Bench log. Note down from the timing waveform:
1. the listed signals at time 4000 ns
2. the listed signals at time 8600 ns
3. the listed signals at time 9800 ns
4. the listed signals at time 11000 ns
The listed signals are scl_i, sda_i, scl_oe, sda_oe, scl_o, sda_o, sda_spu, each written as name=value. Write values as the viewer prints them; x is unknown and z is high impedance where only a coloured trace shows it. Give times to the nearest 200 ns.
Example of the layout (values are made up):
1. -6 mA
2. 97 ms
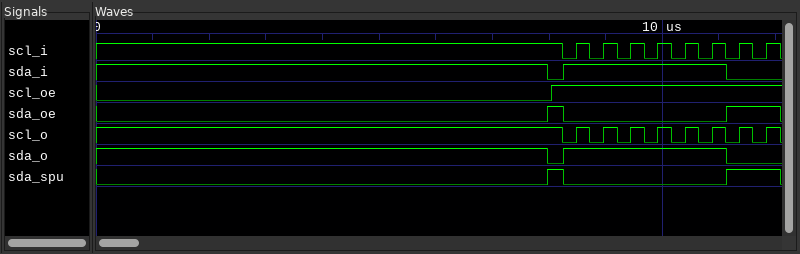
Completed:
1. scl_i=1, sda_i=1, scl_oe=0, sda_oe=0, scl_o=1, sda_o=1, sda_spu=0
2. scl_i=1, sda_i=1, scl_oe=1, sda_oe=0, scl_o=1, sda_o=1, sda_spu=0
3. scl_i=0, sda_i=1, scl_oe=1, sda_oe=0, scl_o=0, sda_o=1, sda_spu=0
4. scl_i=1, sda_i=1, scl_oe=1, sda_oe=0, scl_o=1, sda_o=1, sda_spu=0
